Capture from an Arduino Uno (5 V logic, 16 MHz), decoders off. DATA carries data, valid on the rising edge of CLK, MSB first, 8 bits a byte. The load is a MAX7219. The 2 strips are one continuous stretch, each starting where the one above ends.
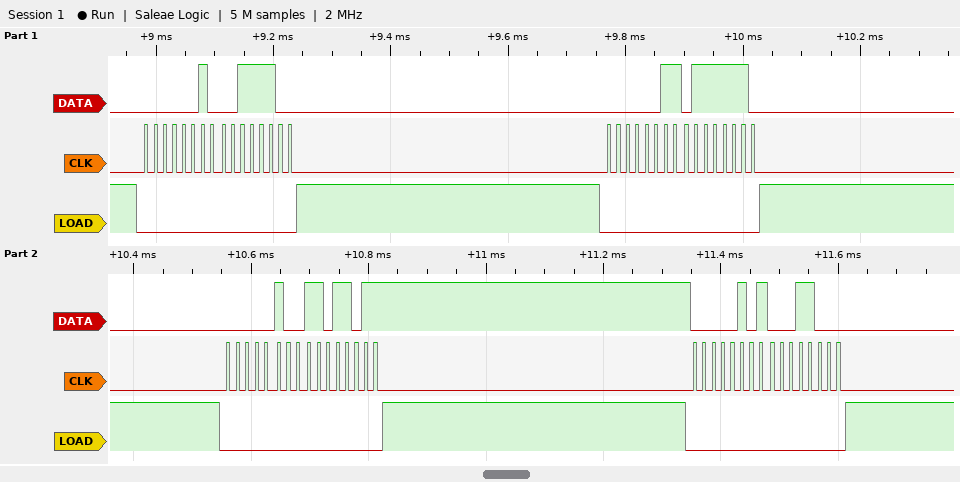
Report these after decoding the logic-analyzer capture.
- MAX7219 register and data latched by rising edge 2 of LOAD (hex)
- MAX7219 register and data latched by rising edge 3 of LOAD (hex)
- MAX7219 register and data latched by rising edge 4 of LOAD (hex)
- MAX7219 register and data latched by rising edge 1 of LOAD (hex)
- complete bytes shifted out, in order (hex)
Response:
register 0x3, data 0x7E
register 0x4, data 0xDB
register 0x5, data 0x18
register 0x2, data 0x3C
02 3C 03 7E 04 DB 05 18
